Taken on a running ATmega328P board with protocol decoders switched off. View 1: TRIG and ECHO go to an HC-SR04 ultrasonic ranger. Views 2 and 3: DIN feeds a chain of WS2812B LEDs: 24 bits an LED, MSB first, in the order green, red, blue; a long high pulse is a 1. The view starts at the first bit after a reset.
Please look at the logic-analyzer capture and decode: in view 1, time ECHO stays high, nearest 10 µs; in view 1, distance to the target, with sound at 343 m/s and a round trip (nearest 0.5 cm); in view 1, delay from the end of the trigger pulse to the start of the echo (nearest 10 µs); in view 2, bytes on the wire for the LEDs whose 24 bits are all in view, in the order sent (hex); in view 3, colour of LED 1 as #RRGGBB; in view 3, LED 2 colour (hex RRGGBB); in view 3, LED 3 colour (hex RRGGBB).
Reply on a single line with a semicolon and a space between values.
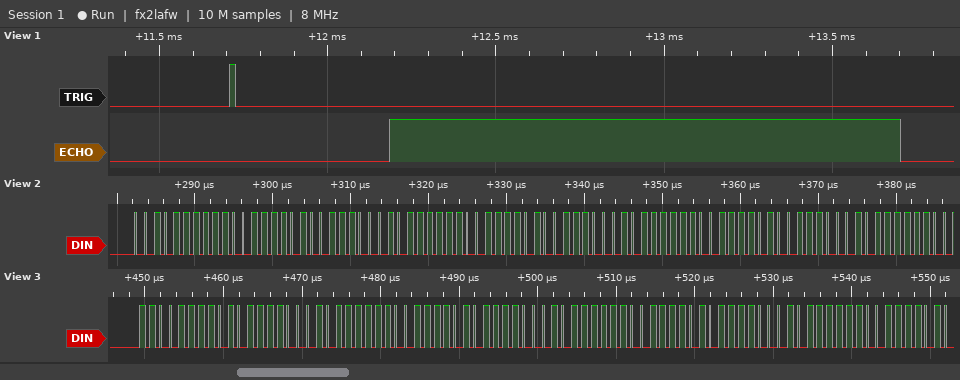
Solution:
1520 µs; 26 cm; 460 µs; 2F CF 4E 2F CF 4E 2F CF 4E; #5ECF2F; #5ECF2F; #5ECF2F
